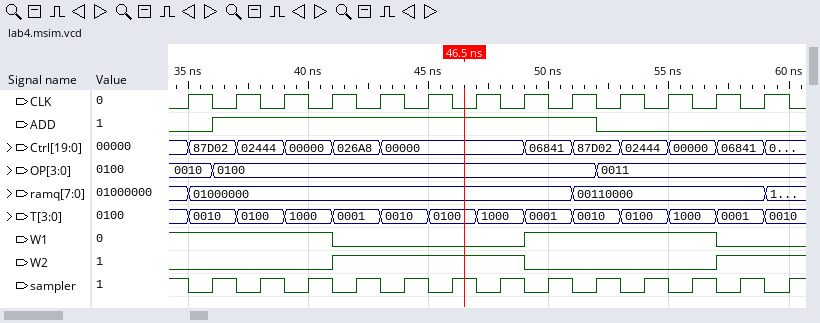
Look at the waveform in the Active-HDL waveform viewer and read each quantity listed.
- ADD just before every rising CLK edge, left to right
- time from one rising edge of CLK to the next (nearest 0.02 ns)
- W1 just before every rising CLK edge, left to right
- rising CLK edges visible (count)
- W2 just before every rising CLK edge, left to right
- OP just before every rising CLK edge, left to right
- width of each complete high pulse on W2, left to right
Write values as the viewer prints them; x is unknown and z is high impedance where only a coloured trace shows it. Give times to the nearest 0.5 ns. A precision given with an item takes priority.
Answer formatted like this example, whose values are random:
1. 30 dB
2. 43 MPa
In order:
1. 0 1 1 1 1 1 1 1 1 0 0 0 0
2. 2 ns
3. 1 1 1 1 0 0 0 0 1 1 1 1 0
4. 13
5. 0 0 0 0 1 1 1 1 0 0 0 0 1
6. 0010, 0100, 0100, 0100, 0100, 0100, 0100, 0100, 0100, 0011, 0011, 0011, 0011
7. 8 ns
